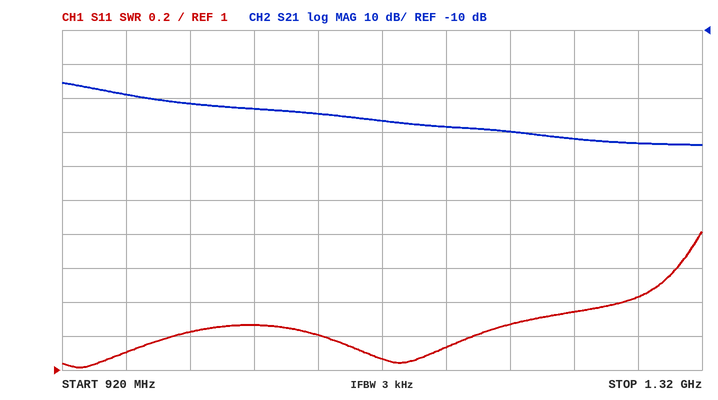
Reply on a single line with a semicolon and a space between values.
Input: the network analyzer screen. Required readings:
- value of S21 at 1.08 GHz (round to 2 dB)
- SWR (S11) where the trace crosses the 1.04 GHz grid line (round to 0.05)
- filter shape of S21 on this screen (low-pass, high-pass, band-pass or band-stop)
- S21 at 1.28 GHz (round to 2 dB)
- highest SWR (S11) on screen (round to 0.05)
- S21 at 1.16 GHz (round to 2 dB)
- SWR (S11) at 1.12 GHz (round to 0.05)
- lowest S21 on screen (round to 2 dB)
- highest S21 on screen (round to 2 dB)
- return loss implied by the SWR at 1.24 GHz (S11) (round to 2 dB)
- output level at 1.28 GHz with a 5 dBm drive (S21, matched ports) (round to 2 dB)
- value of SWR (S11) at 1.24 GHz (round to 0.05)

-34 dB; 1.25; low-pass; -44 dB; 1.80; -38 dB; 1.05; -44 dB; -26 dB; 16 dB; -38 dBm; 1.35
